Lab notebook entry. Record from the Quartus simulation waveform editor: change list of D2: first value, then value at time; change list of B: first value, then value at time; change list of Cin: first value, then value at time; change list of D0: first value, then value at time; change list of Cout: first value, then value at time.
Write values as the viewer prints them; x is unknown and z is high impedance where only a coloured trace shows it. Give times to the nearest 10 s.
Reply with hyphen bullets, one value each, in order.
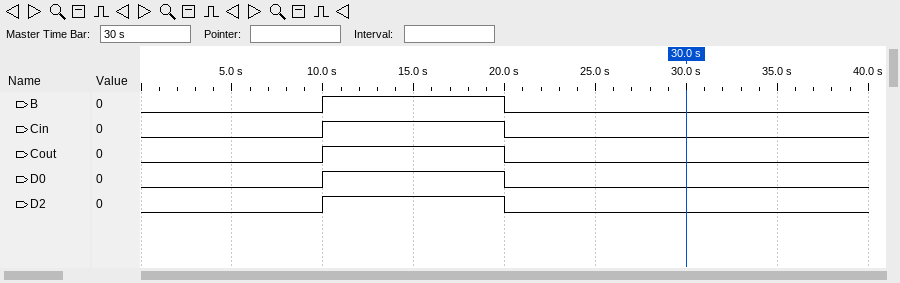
- 0, 1 at 10 s, 0 at 20 s
- 0, 1 at 10 s, 0 at 20 s
- 0, 1 at 10 s, 0 at 20 s
- 0, 1 at 10 s, 0 at 20 s
- 0, 1 at 10 s, 0 at 20 s
